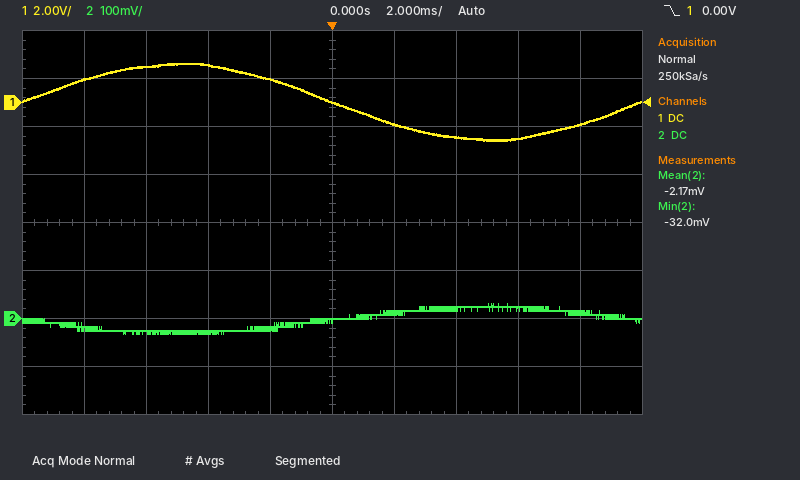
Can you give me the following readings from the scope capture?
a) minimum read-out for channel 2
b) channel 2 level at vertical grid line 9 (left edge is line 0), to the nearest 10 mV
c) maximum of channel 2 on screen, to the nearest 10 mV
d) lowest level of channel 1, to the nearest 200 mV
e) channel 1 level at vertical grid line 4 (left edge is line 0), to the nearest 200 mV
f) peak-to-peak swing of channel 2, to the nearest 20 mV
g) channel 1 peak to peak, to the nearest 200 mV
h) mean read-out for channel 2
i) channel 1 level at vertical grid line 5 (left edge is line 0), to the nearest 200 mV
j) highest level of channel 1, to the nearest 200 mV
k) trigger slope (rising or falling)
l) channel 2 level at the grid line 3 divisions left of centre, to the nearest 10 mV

-32.0 mV
10 mV
30 mV
-1.6 V
1.0 V
60 mV
3.2 V
-2.17 mV
0.0 V
1.6 V
falling
-30 mV
